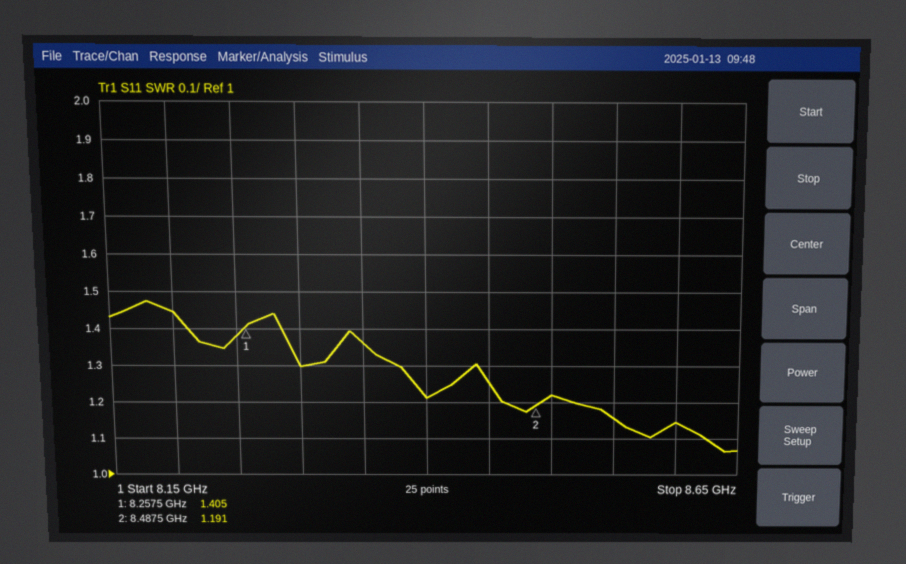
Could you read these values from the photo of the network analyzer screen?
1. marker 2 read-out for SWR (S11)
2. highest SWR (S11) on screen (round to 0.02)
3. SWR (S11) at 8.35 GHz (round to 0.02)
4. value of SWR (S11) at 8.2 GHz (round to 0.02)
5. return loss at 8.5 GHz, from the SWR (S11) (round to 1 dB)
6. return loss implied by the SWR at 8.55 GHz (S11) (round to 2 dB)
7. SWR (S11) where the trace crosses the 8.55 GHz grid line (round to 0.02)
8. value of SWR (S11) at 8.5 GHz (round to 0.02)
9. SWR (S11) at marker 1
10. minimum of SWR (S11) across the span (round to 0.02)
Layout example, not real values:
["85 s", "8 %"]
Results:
["1.191", "1.48", "1.36", "1.44", "20 dB", "22 dB", "1.16", "1.22", "1.405", "1.06"]
